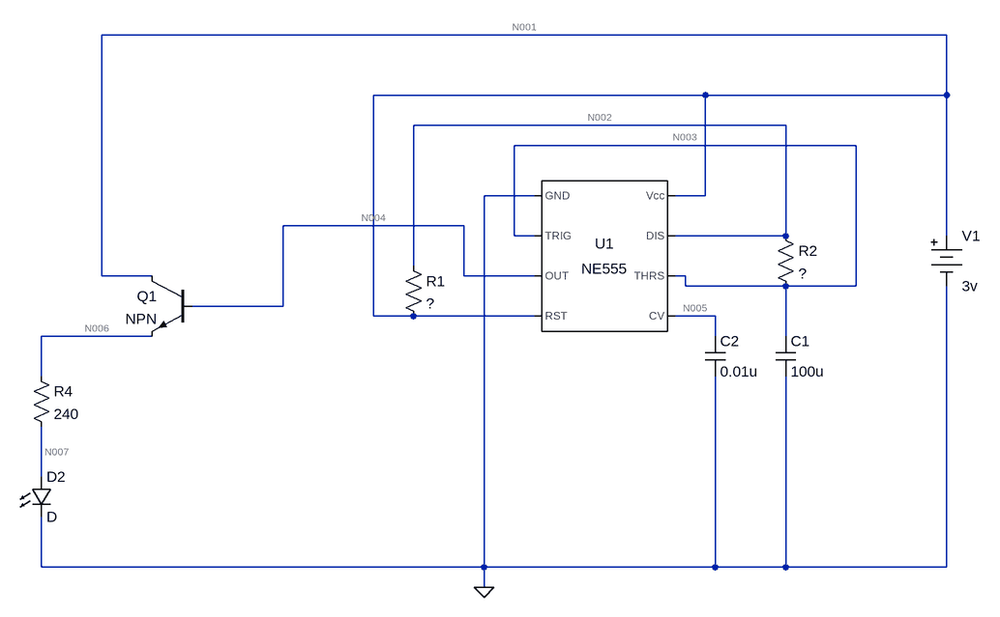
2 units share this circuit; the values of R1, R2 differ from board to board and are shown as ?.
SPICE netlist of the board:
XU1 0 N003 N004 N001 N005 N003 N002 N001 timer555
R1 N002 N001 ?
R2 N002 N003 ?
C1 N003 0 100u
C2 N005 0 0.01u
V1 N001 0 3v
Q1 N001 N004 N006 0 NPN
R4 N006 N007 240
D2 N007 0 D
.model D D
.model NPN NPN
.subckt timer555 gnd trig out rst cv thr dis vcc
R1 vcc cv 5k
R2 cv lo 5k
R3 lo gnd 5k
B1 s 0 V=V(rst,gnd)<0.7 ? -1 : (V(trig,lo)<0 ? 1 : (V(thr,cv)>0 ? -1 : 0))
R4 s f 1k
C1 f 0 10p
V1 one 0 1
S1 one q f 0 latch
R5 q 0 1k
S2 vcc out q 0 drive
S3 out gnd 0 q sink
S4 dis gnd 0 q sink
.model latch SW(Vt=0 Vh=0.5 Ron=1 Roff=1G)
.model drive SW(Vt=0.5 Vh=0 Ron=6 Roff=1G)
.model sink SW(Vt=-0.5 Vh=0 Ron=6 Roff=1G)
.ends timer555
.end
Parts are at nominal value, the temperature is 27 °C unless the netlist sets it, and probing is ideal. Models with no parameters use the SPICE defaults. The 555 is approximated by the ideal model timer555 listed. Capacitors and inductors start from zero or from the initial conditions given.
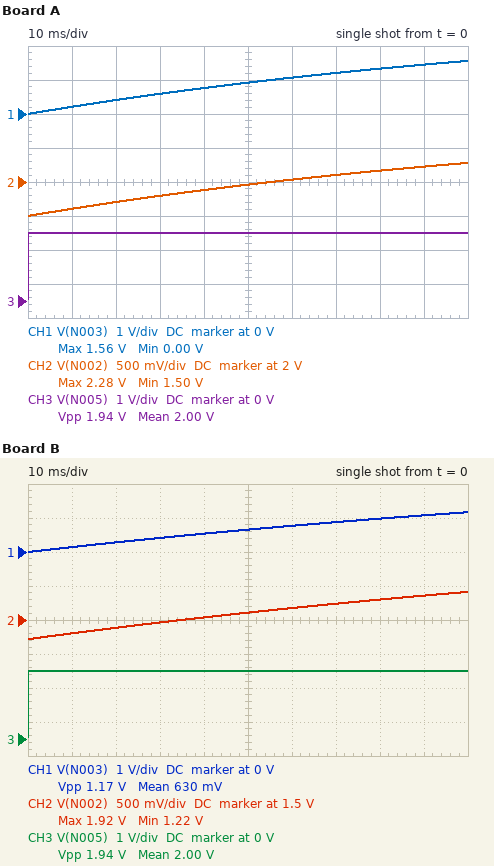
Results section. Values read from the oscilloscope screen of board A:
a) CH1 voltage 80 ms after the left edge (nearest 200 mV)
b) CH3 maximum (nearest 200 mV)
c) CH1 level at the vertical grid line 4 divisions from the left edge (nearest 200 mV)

1.4 V
2.0 V
800 mV
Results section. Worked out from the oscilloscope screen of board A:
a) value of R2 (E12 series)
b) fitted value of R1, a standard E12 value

680 Ω
680 Ω
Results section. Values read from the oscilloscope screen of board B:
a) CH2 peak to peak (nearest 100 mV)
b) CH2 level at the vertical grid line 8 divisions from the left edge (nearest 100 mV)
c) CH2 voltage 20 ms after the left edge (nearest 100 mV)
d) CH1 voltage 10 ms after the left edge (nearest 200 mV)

700 mV
1.8 V
1.4 V
200 mV
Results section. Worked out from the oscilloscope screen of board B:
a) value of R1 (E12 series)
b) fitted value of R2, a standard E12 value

1.2 kΩ
820 Ω
